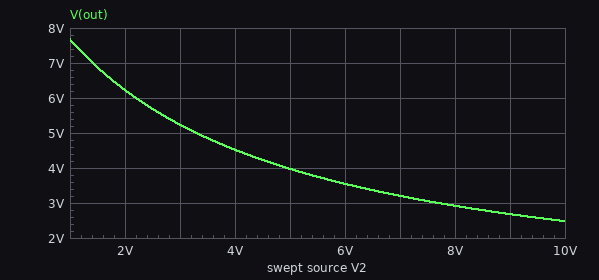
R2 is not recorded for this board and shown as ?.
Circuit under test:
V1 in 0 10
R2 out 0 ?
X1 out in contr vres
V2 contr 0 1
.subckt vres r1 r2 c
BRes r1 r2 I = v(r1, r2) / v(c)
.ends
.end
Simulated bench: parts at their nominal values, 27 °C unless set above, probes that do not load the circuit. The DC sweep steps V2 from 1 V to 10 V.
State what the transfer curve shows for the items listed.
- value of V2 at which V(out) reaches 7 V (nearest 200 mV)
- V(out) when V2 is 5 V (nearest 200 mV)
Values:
1.4 V
4.0 V
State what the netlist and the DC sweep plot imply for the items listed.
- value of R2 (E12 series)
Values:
3.3 Ω
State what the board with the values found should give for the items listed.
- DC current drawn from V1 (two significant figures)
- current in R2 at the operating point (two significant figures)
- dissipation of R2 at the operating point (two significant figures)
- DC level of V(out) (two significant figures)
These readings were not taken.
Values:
2.3 A
2.3 A
18 W
7.7 V
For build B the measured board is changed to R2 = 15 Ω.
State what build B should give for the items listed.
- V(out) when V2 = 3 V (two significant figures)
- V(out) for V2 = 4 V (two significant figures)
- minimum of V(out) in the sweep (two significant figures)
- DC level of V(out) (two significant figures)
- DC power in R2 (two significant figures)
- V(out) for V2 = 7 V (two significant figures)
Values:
8.3 V
7.9 V
6.0 V
9.4 V
5.9 W
6.8 V
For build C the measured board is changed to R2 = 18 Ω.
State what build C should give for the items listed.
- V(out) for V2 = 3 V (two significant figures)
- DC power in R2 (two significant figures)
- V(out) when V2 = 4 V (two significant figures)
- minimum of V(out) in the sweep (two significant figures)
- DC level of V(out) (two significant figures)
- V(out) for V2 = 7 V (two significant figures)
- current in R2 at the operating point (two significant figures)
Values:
8.6 V
5.0 W
8.2 V
6.4 V
9.5 V
7.2 V
530 mA
